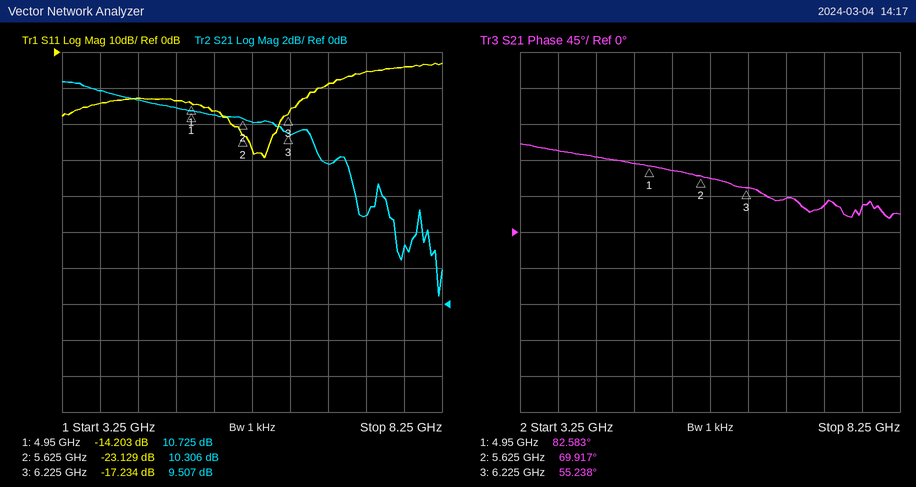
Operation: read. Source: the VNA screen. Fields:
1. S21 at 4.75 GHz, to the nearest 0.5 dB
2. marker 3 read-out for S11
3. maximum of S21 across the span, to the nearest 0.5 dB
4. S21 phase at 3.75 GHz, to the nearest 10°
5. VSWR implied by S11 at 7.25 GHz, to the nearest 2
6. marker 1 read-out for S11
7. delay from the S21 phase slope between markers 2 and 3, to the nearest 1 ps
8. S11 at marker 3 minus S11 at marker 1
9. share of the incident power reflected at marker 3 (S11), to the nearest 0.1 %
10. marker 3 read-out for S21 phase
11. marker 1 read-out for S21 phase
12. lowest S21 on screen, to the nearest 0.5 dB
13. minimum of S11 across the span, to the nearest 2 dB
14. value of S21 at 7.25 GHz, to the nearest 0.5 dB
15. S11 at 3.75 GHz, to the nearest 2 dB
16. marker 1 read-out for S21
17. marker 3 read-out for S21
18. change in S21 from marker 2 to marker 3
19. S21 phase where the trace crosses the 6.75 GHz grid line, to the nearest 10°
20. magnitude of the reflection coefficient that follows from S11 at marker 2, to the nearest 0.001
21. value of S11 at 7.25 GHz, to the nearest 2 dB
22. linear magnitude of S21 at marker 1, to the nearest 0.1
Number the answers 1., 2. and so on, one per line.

1. 11.0 dB
2. -17.234 dB
3. 12.5 dB
4. 100°
5. 4
6. -14.203 dB
7. 68 ps
8. -3.031 dB
9. 1.9 %
10. 55.238°
11. 82.583°
12. 0.5 dB
13. -30 dB
14. 5.0 dB
15. -14 dB
16. 10.725 dB
17. 9.507 dB
18. -0.799 dB
19. 40°
20. 0.070
21. -6 dB
22. 3.4
